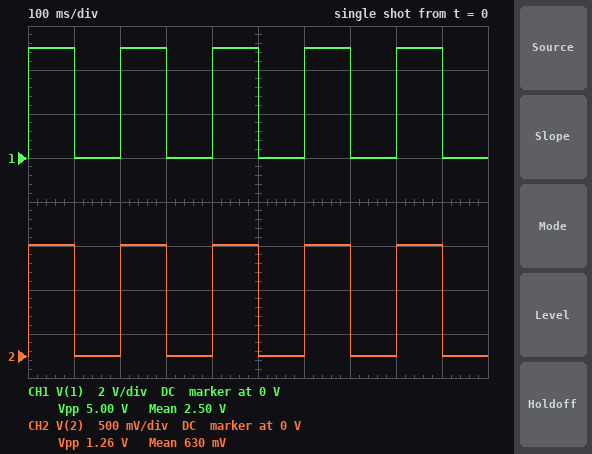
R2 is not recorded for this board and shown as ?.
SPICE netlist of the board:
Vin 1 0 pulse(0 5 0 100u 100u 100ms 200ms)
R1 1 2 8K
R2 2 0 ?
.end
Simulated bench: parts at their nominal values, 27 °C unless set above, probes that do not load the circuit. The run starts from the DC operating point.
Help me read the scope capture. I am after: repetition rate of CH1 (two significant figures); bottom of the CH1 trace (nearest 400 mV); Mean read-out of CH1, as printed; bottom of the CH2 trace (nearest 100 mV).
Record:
5.0 Hz
0 V
2.50 V
0 V
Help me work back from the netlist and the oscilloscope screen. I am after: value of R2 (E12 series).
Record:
2.7 kΩ
